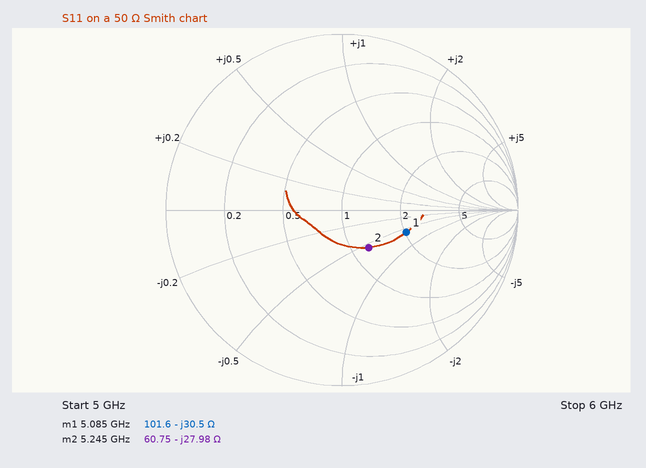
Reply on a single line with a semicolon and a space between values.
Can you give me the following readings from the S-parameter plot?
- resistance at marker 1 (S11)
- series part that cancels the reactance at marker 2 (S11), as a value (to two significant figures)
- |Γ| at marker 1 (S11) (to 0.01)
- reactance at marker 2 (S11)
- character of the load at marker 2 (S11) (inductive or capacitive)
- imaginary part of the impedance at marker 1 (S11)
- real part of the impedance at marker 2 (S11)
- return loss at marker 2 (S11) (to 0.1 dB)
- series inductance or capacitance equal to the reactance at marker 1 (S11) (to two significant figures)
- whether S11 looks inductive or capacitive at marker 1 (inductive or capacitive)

101.6 Ω; 850 pH; 0.39; -27.98 Ω; capacitive; -30.5 Ω; 60.75 Ω; 11.6 dB; 1.0 pF; capacitive
